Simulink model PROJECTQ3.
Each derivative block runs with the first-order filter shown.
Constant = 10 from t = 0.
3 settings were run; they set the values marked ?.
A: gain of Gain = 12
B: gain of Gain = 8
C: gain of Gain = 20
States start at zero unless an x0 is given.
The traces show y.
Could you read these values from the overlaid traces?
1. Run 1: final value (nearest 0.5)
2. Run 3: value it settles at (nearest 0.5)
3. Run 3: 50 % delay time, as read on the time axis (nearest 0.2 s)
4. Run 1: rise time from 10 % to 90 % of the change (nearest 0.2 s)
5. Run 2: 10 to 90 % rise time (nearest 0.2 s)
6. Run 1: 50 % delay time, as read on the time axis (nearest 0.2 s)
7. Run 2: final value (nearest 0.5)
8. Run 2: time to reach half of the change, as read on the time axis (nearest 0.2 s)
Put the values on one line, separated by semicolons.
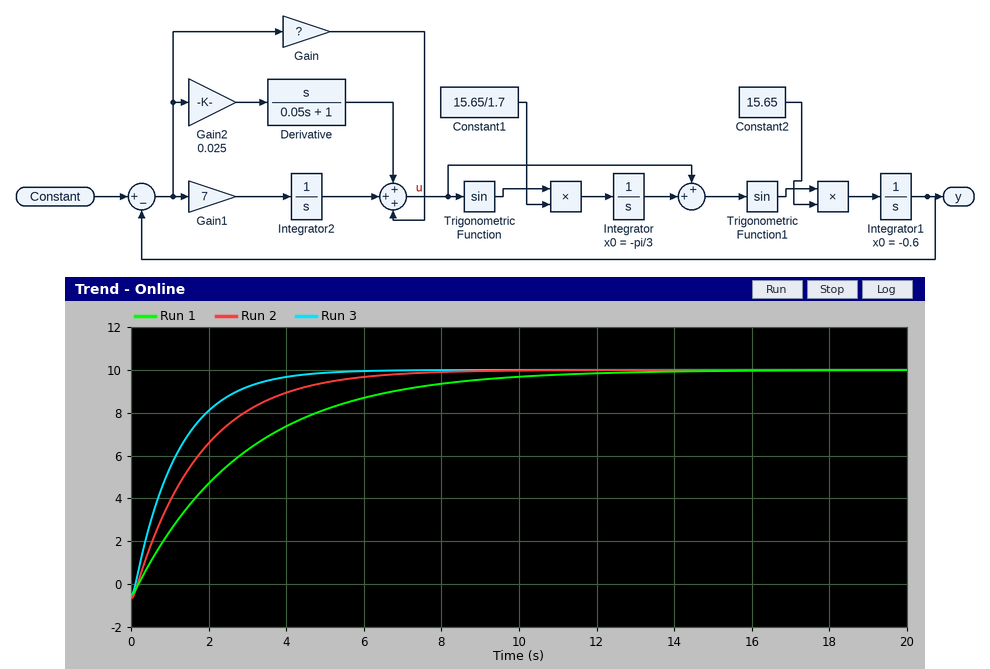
10.0; 10.0; 0.8 s; 6.2 s; 3.8 s; 2.0 s; 10.0; 1.2 s
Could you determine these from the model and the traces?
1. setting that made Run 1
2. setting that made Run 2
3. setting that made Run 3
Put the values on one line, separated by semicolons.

C; A; B
